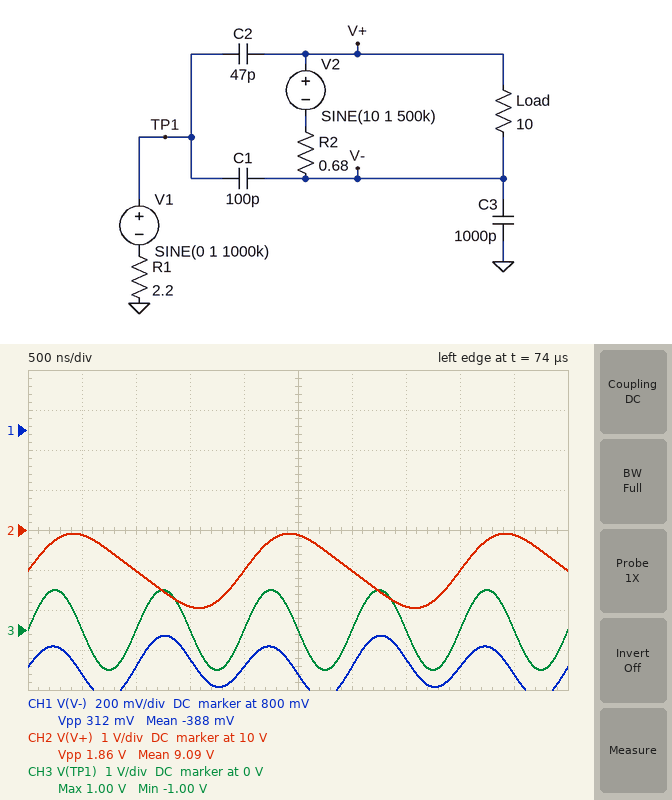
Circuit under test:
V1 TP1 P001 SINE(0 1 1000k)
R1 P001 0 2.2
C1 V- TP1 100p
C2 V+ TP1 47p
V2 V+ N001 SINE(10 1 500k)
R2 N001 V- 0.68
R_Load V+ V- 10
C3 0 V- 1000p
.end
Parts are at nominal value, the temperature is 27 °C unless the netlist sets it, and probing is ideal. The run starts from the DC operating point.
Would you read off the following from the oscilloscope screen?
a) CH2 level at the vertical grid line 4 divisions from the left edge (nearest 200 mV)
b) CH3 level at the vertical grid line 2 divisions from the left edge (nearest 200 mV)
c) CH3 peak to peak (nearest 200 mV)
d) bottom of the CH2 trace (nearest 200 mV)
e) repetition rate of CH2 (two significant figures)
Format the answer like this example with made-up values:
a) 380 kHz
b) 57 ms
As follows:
a) 9.0 V
b) 0 V
c) 2.0 V
d) 8.0 V
e) 500 kHz
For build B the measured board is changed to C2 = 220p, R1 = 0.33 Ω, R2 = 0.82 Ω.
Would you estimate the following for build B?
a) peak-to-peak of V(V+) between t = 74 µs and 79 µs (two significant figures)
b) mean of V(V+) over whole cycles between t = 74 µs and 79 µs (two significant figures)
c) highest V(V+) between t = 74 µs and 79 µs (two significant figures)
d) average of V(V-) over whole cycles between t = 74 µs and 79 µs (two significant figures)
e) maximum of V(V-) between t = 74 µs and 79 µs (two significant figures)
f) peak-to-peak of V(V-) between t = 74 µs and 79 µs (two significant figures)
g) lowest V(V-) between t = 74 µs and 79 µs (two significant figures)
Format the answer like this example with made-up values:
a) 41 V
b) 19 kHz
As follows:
a) 1.8 V
b) 7.7 V
c) 8.6 V
d) -1.5 V
e) -1.2 V
f) 710 mV
g) -1.9 V
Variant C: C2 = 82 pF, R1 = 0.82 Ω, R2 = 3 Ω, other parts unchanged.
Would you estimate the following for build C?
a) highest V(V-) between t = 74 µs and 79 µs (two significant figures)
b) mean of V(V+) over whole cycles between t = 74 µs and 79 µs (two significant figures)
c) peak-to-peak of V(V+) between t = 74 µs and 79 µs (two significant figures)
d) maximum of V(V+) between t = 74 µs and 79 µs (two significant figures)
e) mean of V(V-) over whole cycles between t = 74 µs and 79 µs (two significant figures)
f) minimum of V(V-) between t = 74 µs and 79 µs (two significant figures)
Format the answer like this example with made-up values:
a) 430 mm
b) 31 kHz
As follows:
a) -340 mV
b) 7.2 V
c) 1.5 V
d) 7.9 V
e) -540 mV
f) -730 mV
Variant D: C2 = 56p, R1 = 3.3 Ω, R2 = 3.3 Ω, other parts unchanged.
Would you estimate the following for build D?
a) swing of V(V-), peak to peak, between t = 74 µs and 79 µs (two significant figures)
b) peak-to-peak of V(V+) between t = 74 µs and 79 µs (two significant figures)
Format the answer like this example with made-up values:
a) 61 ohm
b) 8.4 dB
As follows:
a) 320 mV
b) 1.5 V
